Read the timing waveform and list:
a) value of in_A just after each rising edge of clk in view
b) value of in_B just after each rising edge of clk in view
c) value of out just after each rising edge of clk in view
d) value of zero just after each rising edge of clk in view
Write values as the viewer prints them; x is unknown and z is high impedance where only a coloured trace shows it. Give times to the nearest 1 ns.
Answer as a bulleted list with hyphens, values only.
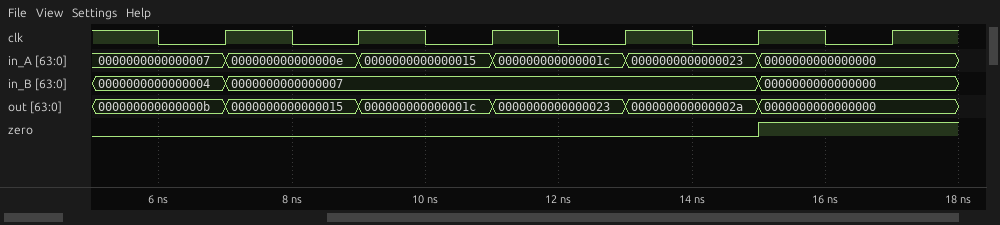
- 000000000000000e, 0000000000000015, 000000000000001c, 0000000000000023, 0000000000000000, 0000000000000000
- 0000000000000007, 0000000000000007, 0000000000000007, 0000000000000007, 0000000000000000, 0000000000000000
- 0000000000000015, 000000000000001c, 0000000000000023, 000000000000002a, 0000000000000000, 0000000000000000
- 0 0 0 0 1 1
